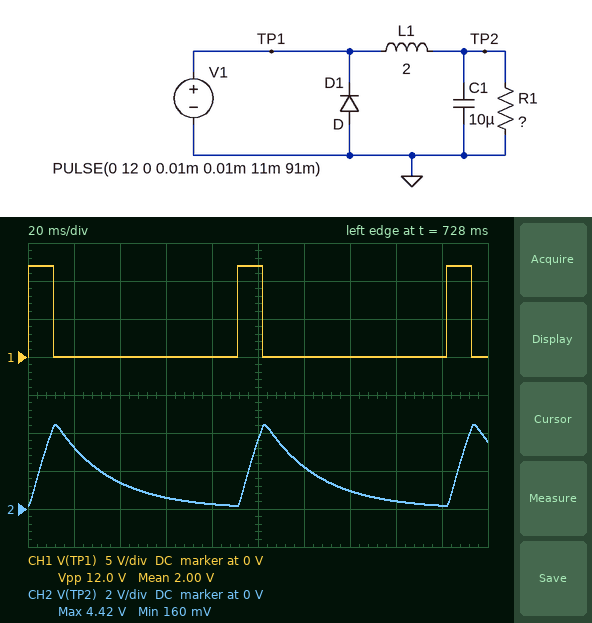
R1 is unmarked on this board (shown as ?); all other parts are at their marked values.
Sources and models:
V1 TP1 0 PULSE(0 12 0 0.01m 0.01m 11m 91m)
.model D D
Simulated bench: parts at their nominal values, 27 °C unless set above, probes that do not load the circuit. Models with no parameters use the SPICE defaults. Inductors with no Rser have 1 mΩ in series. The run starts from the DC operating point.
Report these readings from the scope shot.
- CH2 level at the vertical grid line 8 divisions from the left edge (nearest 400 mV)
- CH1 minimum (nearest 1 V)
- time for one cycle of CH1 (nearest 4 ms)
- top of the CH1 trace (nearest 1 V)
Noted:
400 mV
0 V
92 ms
12 V
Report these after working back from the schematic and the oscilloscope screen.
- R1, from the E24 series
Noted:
82 Ω
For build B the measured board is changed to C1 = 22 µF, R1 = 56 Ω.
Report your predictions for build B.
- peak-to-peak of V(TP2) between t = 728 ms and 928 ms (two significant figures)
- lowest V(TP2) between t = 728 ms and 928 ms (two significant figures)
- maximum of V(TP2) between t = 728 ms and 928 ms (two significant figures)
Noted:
3.0 V
360 mV
3.4 V
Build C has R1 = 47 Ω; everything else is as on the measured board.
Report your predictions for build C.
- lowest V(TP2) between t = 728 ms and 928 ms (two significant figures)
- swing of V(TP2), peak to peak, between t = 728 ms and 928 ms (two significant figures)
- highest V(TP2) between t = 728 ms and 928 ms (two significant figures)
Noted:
470 mV
2.6 V
3.1 V
